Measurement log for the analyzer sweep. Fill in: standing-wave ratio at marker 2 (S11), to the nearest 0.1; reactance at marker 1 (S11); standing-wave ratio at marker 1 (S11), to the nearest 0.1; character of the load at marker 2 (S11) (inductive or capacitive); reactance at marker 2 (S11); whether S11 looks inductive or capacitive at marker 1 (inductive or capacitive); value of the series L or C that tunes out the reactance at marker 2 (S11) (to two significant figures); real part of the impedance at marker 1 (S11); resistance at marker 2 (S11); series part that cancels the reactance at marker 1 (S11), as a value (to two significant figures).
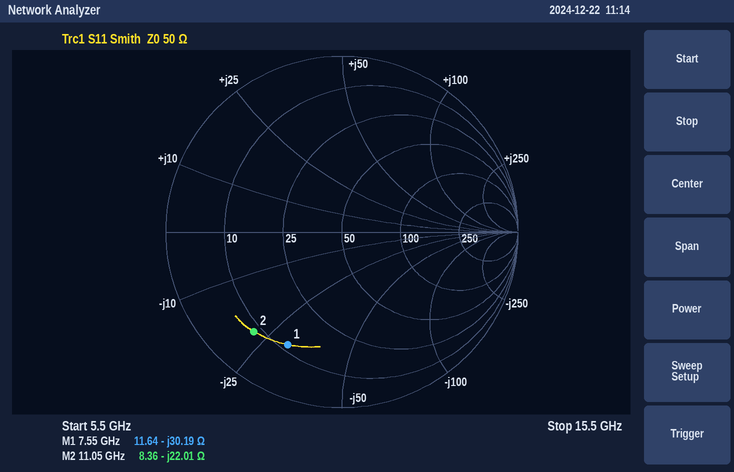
7.2
-30.19 Ω
5.9
capacitive
-22.01 Ω
capacitive
320 pH
11.64 Ω
8.36 Ω
640 pH
